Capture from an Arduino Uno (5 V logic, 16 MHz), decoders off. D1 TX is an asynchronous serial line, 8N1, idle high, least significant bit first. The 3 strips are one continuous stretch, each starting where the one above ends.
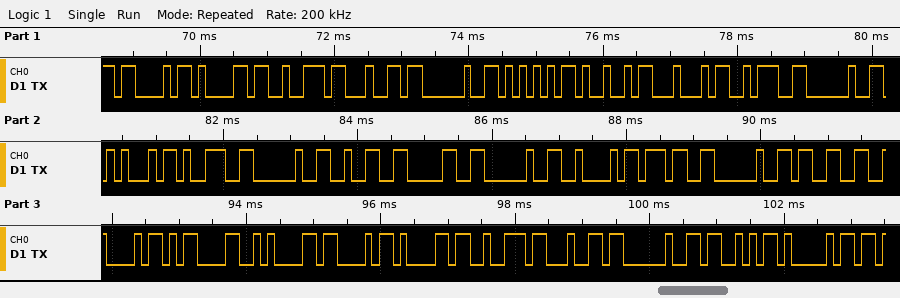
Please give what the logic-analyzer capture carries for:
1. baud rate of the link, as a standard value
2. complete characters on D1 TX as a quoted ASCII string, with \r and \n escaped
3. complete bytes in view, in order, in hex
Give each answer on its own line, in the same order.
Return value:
9600 baud
"Card UID: E9 20 B7 3B\r\nCard SA"
43 61 72 64 20 55 49 44 3A 20 45 39 20 32 30 20 42 37 20 33 42 0D 0A 43 61 72 64 20 53 41
